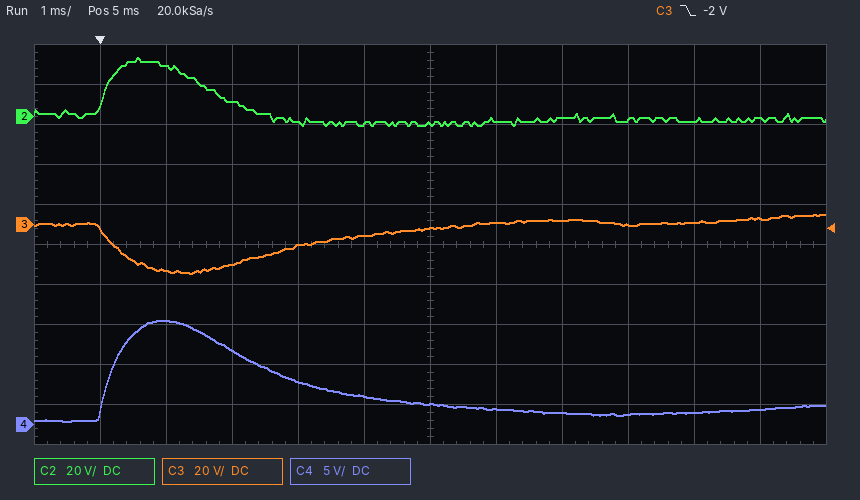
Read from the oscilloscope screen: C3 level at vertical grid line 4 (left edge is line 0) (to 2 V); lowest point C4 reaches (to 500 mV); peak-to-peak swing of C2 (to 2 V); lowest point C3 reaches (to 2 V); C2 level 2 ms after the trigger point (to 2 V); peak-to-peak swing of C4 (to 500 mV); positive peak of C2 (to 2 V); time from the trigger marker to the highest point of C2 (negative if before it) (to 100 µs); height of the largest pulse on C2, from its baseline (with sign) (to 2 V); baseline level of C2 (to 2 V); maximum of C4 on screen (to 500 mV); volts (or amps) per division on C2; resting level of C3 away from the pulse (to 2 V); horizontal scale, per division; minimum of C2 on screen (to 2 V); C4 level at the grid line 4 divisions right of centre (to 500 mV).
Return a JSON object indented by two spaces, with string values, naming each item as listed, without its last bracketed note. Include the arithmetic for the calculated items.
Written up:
{
  "C3 level at vertical grid line 4 (left edge is line 0)": "-10 V",
  "lowest point C4 reaches": "500 mV",
  "peak-to-peak swing of C2": "30 V − (-4 V) = 34 V",
  "lowest point C3 reaches": "-24 V",
  "C2 level 2 ms after the trigger point": "8 V",
  "peak-to-peak swing of C4": "13.0 V − (500 mV) = 12.5 V",
  "positive peak of C2": "30 V",
  "time from the trigger marker to the highest point of C2 (negative if before it)": "+600 µs",
  "height of the largest pulse on C2, from its baseline (with sign)": "30 V − (-2 V) = +32 V",
  "baseline level of C2": "-2 V",
  "maximum of C4 on screen": "13.0 V",
  "volts (or amps) per division on C2": "20 V",
  "resting level of C3 away from the pulse": "0 V",
  "horizontal scale, per division": "1 ms",
  "minimum of C2 on screen": "-4 V",
  "C4 level at the grid line 4 divisions right of centre": "1.5 V"
}
